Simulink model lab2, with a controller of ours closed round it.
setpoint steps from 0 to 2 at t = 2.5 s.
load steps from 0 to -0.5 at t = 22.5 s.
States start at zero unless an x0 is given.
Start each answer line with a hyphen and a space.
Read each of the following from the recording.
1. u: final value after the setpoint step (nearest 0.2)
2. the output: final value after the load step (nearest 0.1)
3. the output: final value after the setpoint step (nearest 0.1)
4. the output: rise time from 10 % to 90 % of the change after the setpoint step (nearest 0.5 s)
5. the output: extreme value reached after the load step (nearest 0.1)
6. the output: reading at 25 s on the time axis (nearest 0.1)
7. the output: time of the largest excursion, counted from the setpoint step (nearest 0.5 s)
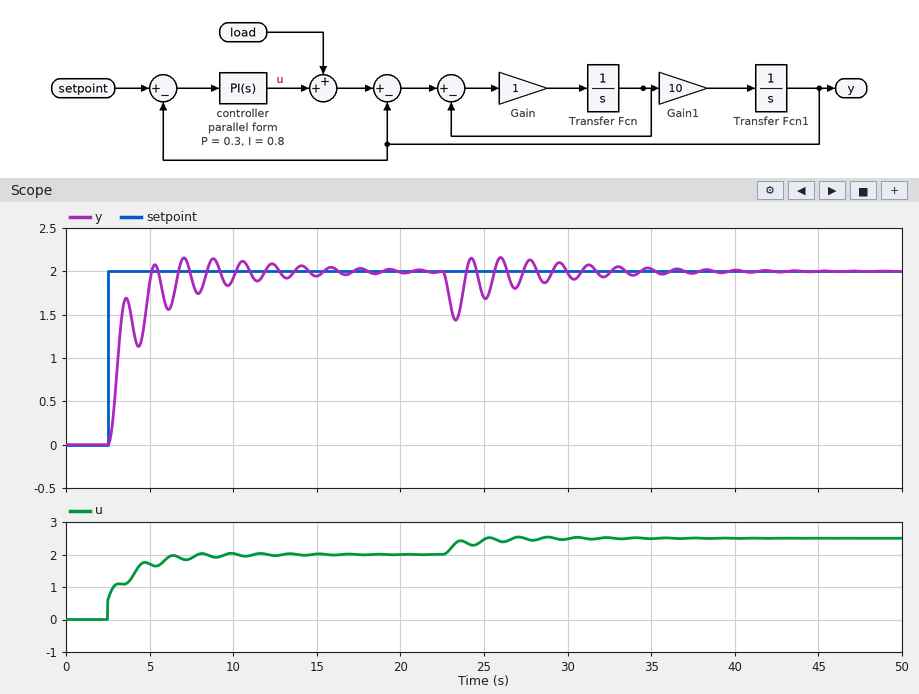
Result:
- 2.0
- 2.0
- 2.0
- 2.0 s
- 1.4
- 1.7
- 4.5 s
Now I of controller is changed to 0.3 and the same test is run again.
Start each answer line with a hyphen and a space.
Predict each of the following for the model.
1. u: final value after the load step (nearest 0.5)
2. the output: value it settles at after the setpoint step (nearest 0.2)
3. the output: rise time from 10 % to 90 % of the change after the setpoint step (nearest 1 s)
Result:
- 2.5
- 2.0
- 9 s
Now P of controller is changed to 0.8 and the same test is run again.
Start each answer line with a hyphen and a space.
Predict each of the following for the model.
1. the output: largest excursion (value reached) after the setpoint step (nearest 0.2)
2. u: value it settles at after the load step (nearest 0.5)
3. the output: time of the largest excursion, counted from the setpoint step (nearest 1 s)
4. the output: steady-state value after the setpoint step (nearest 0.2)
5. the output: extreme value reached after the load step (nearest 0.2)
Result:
- 2.2
- 2.5
- 4 s
- 2.0
- 1.6
